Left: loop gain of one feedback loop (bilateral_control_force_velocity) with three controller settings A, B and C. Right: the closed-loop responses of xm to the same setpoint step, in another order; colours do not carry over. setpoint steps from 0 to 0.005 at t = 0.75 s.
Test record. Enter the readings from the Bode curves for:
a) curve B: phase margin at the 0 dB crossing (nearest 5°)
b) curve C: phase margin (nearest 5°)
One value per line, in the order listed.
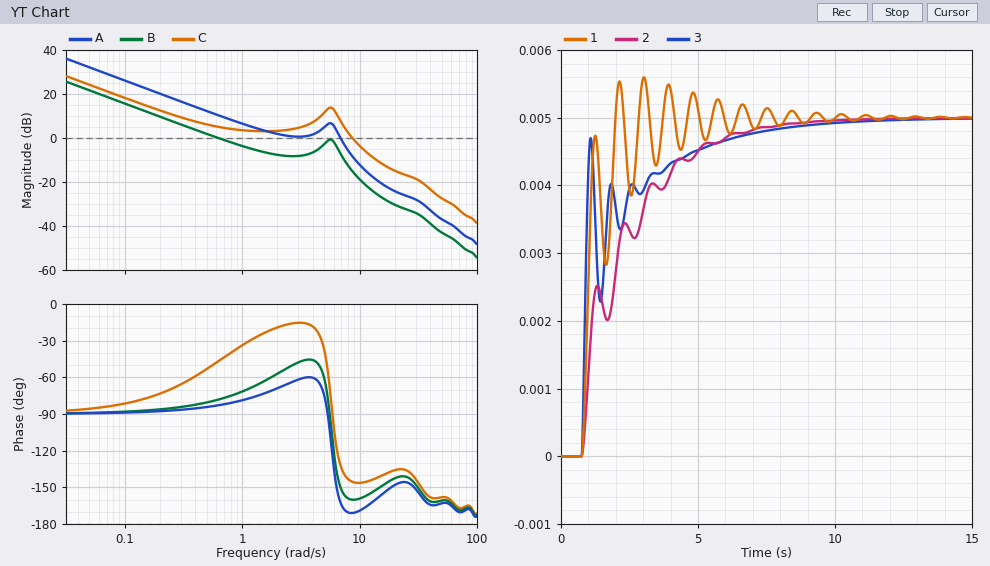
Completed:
100°
35°
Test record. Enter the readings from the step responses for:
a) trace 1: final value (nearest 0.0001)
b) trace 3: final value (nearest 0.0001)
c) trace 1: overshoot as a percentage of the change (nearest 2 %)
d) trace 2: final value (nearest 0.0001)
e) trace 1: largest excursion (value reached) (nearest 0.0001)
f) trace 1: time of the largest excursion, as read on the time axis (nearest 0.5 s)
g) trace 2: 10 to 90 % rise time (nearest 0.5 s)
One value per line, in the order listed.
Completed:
0.0050
0.0050
12 %
0.0050
0.0056
3.0 s
4.0 s
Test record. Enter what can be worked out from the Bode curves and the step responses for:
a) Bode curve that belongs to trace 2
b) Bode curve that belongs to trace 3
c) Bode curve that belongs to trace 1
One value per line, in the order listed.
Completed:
B
C
A
